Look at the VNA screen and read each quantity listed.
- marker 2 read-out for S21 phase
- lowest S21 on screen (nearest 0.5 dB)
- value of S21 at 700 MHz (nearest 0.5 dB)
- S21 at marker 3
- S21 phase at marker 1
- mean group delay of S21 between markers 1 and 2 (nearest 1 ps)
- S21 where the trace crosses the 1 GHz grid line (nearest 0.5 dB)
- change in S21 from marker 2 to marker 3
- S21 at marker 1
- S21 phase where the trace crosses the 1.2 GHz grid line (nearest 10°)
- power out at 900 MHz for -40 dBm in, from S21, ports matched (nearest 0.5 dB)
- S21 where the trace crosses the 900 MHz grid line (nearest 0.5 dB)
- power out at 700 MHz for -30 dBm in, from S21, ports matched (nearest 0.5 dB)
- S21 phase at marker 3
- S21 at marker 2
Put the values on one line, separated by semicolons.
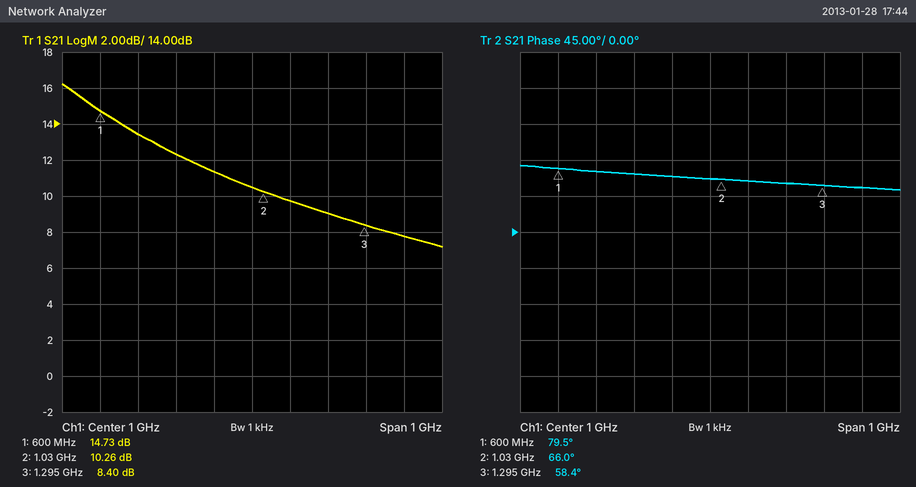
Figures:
66.0°; 7.0 dB; 13.5 dB; 8.40 dB; 79.5°; 87 ps; 10.5 dB; -1.86 dB; 14.73 dB; 60°; -28.5 dBm; 11.5 dB; -16.5 dBm; 58.4°; 10.26 dB
